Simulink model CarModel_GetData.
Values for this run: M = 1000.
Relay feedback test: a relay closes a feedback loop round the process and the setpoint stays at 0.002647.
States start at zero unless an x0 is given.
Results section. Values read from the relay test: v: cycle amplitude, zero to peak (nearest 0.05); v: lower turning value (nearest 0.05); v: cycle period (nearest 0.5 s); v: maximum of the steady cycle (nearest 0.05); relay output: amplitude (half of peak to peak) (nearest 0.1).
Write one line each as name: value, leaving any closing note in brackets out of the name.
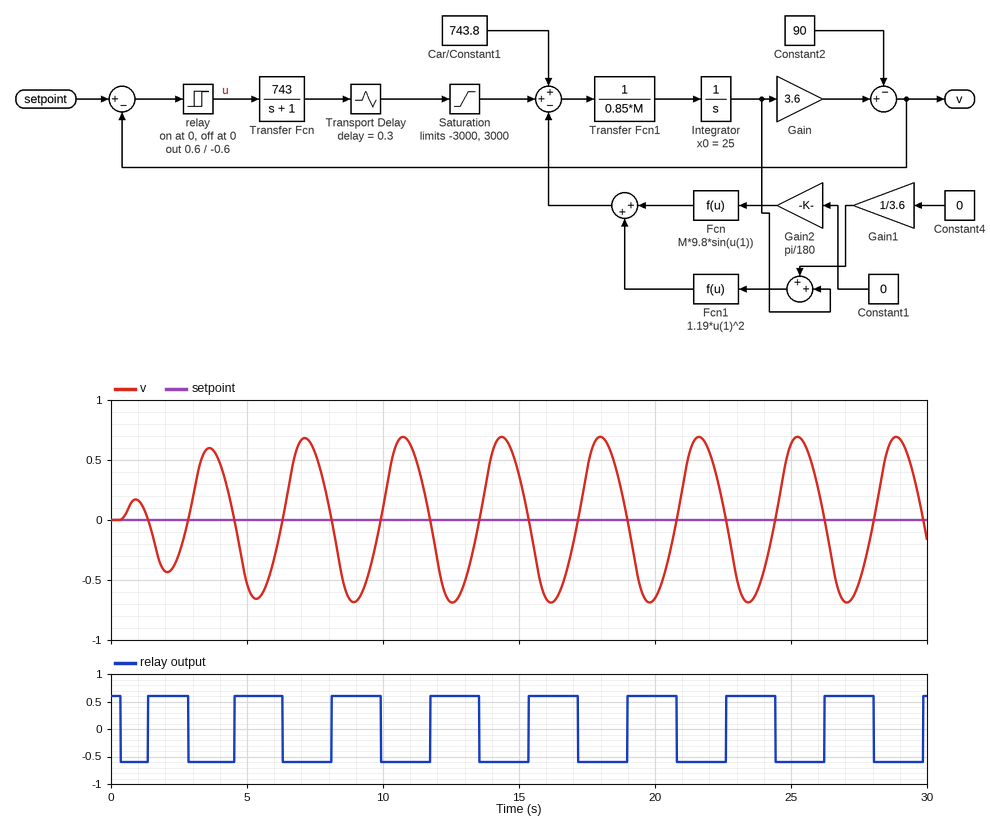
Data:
v: cycle amplitude, zero to peak: 0.70
v: lower turning value: -0.70
v: cycle period: 3.5 s
v: maximum of the steady cycle: 0.70
relay output: amplitude (half of peak to peak): 0.6
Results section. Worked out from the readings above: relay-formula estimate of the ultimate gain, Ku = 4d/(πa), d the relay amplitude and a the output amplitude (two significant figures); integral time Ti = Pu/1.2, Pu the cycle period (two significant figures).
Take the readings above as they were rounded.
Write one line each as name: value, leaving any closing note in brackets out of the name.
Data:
relay-formula estimate of the ultimate gain, Ku = 4d/(πa), d the relay amplitude and a the output amplitude: 1.1
integral time Ti = Pu/1.2, Pu the cycle period: 2.9 s
